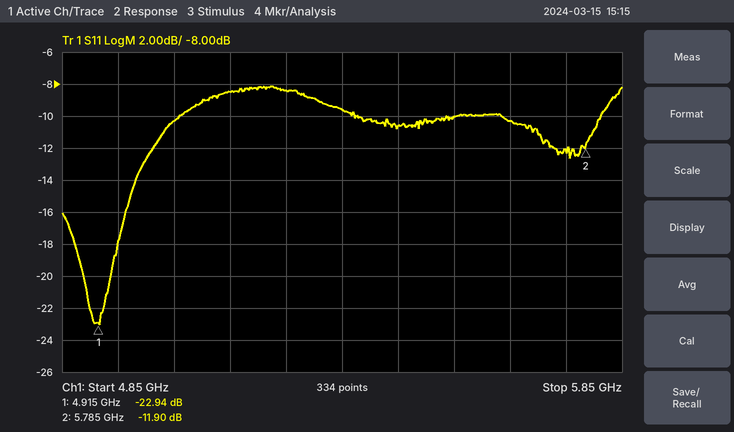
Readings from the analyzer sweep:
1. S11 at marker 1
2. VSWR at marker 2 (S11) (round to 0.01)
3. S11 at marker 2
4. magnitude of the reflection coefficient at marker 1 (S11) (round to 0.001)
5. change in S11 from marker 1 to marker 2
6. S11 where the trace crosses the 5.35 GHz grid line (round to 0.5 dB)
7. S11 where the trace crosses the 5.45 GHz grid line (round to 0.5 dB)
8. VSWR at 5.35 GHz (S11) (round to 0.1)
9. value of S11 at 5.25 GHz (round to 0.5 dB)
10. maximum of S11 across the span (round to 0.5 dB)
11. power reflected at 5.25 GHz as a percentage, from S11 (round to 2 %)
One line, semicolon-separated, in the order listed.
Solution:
-22.94 dB; 1.68; -11.90 dB; 0.071; 11.04 dB; -9.5 dB; -10.5 dB; 2.0; -8.5 dB; -8.0 dB; 14 %
